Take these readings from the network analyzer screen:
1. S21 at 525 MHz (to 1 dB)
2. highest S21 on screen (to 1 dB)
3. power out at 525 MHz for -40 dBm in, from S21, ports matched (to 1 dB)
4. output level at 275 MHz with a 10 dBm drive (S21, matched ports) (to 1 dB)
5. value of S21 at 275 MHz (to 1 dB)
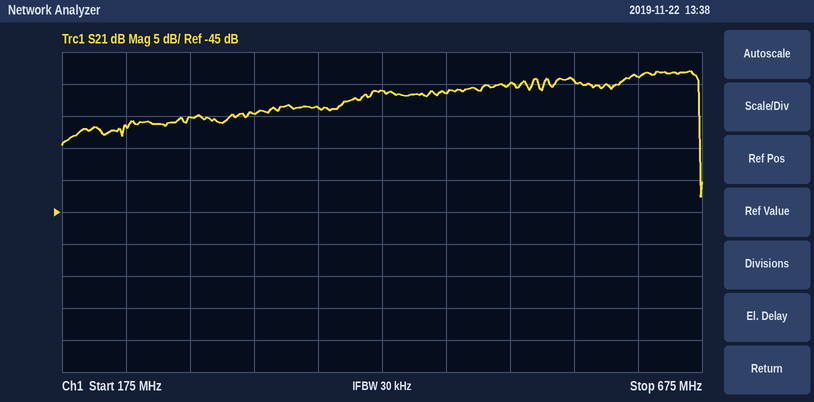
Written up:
-25 dB
-23 dB
-65 dBm
-20 dBm
-30 dB
